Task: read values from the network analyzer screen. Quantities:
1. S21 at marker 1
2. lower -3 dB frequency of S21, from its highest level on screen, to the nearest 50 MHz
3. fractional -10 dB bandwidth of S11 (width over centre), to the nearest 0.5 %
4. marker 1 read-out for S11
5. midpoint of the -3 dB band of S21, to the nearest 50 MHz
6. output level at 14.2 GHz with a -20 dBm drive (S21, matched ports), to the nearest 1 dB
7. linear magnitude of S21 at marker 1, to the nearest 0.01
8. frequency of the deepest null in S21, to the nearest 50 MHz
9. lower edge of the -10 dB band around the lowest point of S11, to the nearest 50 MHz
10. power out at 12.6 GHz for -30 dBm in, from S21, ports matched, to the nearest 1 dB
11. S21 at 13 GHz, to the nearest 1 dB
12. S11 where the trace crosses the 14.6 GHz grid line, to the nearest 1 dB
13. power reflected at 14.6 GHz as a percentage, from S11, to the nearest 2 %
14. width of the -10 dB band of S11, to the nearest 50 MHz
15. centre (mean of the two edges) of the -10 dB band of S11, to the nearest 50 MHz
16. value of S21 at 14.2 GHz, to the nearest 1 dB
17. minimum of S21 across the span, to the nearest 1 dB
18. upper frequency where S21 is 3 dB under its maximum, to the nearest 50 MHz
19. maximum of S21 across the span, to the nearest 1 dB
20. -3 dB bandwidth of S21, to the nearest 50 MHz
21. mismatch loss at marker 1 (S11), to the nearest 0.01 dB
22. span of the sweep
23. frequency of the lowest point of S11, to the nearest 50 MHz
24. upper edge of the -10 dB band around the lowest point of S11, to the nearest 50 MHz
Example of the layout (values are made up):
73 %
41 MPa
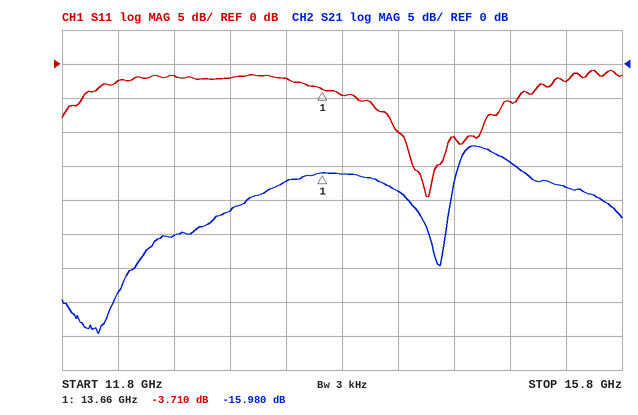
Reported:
-15.980 dB
14.65 GHz
4.0 %
-3.710 dB
14.85 GHz
-39 dBm
0.16
12.05 GHz
14.20 GHz
-55 dBm
-22 dB
-11 dB
8 %
600 MHz
14.50 GHz
-19 dB
-40 dB
15.05 GHz
-12 dB
400 MHz
2.41 dB
4 GHz
14.40 GHz
14.80 GHz
